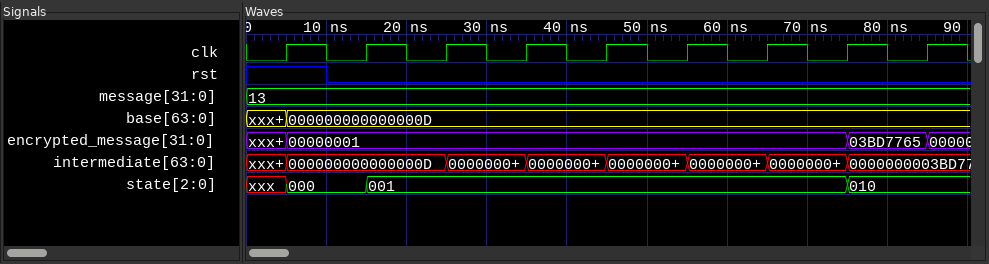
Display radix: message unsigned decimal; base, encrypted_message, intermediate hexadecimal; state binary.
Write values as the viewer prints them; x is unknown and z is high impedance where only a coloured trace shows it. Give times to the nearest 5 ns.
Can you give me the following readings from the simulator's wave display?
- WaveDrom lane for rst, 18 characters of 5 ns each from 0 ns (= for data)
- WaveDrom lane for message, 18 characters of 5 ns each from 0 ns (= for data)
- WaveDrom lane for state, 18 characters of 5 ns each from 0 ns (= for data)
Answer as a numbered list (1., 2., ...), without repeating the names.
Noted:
1. {name: 'rst', wave: '1.0...............'}
2. {name: 'message', wave: '=.................', data: '13'}
3. {name: 'state', wave: 'x=.=...........=..', data: '000 001 010'}
